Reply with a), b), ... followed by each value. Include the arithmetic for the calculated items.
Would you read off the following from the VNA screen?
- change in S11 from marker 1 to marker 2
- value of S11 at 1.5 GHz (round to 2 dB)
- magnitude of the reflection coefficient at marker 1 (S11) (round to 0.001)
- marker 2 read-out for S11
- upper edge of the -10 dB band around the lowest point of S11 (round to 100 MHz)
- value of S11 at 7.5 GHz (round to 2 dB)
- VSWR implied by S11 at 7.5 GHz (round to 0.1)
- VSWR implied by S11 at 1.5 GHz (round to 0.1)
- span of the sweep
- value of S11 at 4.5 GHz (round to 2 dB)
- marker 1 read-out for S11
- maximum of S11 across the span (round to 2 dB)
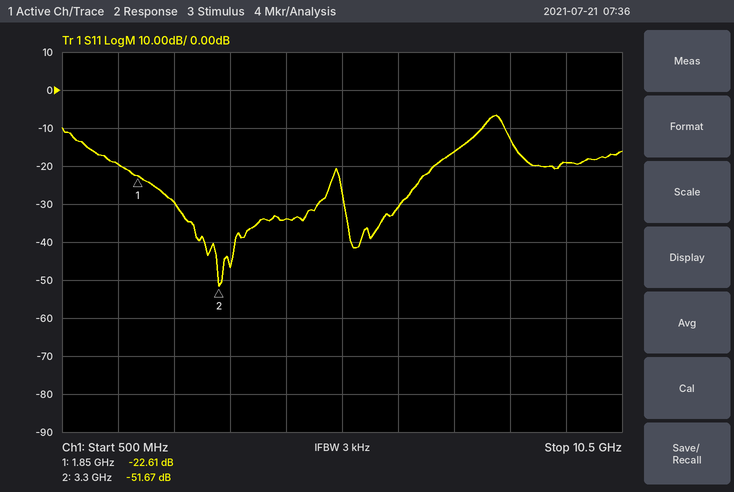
a) -51.67 − (-22.61) = -29.06 dB
b) -20 dB
c) 10^(-22.61/20) ≈ 0.074
d) -51.67 dB
e) 8.0 GHz
f) -16 dB
g) |Γ| = 10^(-16/20) = 0.1585; VSWR = (1 + 0.1585)/(1 − 0.1585) ≈ 1.4
h) |Γ| = 10^(-20/20) = 0.1000; VSWR = (1 + 0.1000)/(1 − 0.1000) ≈ 1.2
i) 10 GHz
j) -34 dB
k) -22.61 dB
l) -6 dB
